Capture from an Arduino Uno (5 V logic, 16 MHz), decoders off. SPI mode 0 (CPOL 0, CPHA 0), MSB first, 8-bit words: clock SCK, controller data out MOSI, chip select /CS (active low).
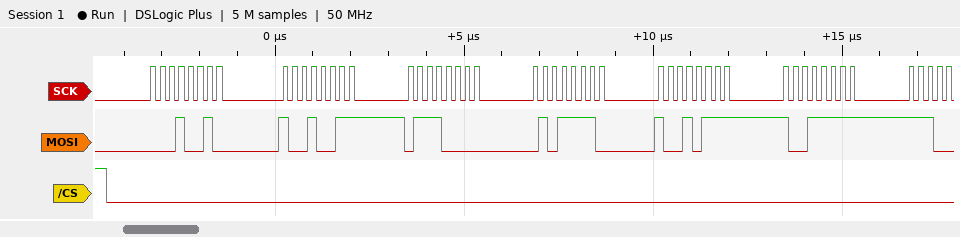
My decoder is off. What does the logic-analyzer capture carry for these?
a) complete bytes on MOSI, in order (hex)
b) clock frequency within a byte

0x12 0x93 0x70 0x5E 0x97 0x9F
4 MHz
